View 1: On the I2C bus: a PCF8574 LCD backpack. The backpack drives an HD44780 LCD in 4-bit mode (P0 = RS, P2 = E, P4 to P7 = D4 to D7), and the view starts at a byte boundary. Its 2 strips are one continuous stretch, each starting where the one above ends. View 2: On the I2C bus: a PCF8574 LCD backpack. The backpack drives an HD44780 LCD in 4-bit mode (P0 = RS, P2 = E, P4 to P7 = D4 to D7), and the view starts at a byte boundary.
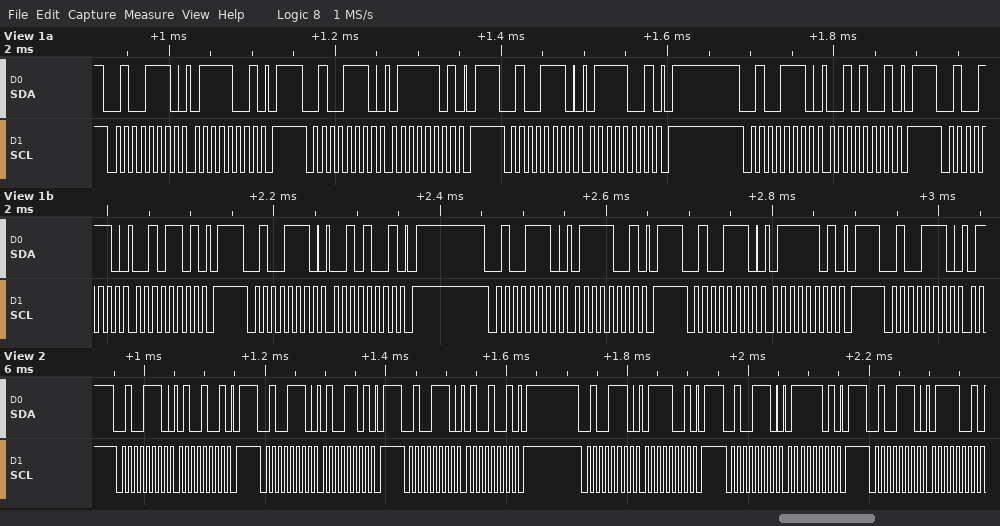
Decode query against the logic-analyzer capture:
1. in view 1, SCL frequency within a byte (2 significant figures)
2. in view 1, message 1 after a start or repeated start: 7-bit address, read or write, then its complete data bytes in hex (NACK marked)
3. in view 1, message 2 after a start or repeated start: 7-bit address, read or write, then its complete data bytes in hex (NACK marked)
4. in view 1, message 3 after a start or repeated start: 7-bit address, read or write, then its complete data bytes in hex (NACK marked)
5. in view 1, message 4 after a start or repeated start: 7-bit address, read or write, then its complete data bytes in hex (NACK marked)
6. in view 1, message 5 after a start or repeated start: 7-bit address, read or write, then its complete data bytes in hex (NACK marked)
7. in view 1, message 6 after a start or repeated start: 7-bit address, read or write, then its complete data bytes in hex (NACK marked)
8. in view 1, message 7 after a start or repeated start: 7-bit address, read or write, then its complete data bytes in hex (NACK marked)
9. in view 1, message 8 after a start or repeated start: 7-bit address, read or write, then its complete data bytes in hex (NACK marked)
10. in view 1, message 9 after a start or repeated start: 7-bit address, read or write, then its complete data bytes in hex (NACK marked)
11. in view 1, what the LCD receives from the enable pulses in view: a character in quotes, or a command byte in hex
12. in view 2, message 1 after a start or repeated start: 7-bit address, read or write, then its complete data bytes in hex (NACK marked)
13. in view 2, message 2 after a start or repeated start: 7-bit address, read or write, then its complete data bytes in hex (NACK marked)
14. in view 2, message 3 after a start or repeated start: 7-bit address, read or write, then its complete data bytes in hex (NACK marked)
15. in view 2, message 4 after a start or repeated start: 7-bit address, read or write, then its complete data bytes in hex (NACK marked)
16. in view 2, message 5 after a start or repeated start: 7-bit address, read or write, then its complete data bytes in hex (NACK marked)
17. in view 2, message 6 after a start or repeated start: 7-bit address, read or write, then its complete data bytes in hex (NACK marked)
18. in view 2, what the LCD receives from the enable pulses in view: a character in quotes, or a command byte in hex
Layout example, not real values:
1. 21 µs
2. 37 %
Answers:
1. 100 kHz
2. 0x27 write: 79
3. 0x27 write: 7D
4. 0x27 write: 79
5. 0x27 write: 29
6. 0x27 write: 2D
7. 0x27 write: 29
8. 0x27 write: 79
9. 0x27 write: 7D
10. 0x27 write
11. 'r'
12. 0x27 write: 49
13. 0x27 write: 4D
14. 0x27 write: 49
15. 0x27 write: 79
16. 0x27 write: 7D
17. 0x27 write: 79
18. 'G'
